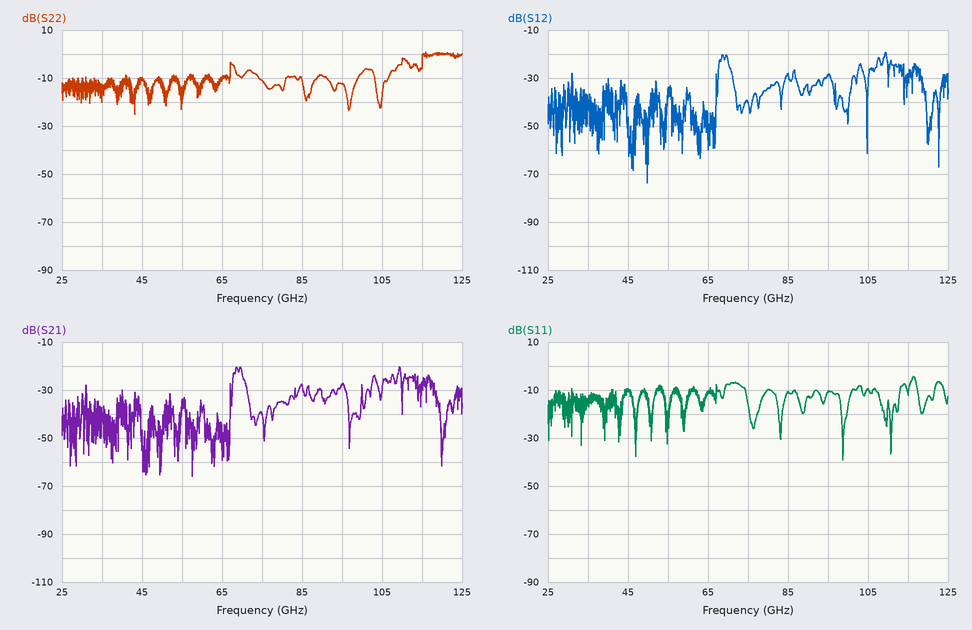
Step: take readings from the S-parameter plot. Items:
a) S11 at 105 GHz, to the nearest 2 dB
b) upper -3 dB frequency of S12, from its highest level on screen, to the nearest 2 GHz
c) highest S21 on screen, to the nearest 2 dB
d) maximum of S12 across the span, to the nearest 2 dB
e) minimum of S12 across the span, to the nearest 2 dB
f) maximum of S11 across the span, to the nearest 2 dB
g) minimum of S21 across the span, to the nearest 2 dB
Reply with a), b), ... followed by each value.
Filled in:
a) -10 dB
b) 110 GHz
c) -20 dB
d) -20 dB
e) -74 dB
f) -4 dB
g) -66 dB
